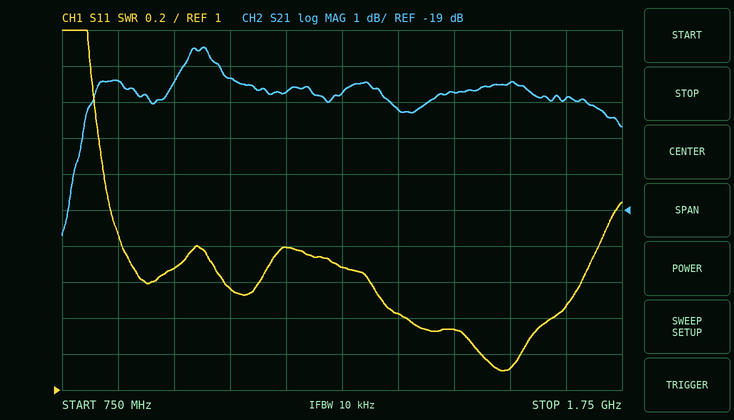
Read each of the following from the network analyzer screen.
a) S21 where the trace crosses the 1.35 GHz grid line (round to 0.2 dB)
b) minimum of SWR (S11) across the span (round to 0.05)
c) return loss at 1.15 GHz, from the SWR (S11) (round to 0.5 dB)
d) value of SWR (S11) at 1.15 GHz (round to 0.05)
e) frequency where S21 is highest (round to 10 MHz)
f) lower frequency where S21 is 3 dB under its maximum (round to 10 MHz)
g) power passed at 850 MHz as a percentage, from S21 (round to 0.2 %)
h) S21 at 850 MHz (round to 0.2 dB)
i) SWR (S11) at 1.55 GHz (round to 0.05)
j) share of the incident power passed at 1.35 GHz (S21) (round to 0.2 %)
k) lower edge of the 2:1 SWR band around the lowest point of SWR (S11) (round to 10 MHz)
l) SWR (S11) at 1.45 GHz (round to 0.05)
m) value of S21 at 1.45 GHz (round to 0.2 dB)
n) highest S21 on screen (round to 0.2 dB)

-16.2 dB
1.10
11.0 dB
1.80
1.00 GHz
780 MHz
2.8 %
-15.4 dB
1.10
2.4 %
840 MHz
1.35
-15.8 dB
-14.4 dB
